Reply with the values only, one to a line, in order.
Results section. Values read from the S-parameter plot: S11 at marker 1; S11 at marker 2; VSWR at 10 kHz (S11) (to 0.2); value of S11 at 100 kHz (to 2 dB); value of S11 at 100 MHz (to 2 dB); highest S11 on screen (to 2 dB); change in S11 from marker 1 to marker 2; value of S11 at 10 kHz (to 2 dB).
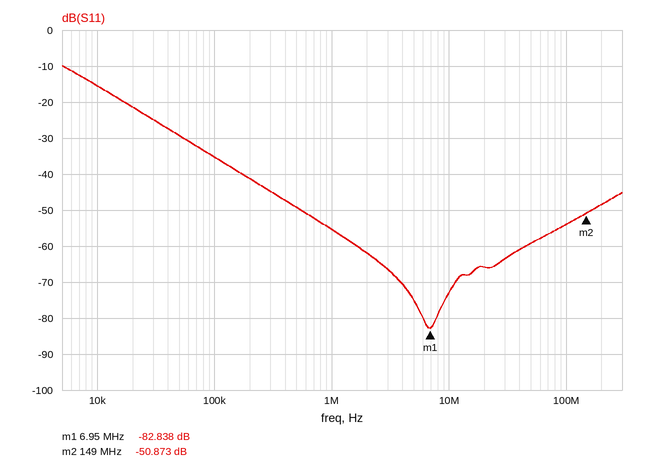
-82.838 dB
-50.873 dB
1.4
-36 dB
-54 dB
-10 dB
31.965 dB
-16 dB
